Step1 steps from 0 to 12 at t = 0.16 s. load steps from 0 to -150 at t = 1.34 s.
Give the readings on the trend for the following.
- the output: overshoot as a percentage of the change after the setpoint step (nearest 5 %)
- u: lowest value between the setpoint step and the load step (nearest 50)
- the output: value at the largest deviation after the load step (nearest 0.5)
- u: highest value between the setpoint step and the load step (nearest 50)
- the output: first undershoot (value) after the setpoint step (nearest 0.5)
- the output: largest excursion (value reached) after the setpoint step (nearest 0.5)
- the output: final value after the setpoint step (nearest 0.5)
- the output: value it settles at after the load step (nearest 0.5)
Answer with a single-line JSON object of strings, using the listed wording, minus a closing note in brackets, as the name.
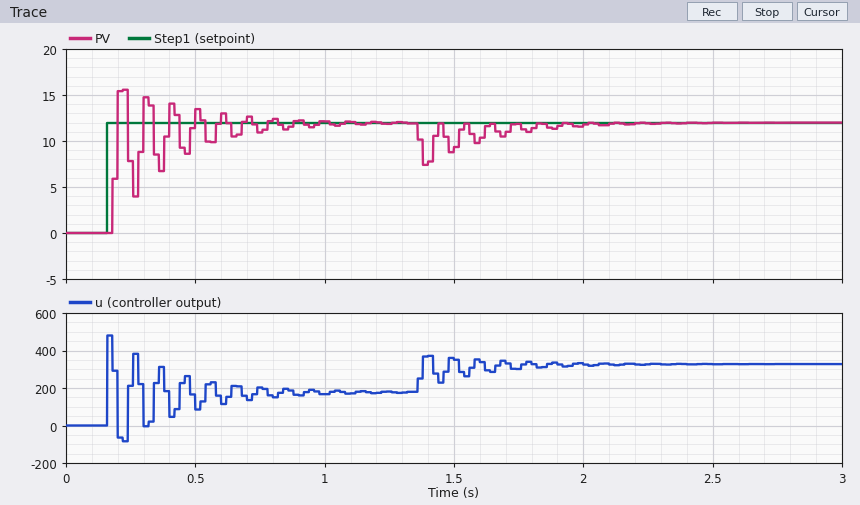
{"the output: overshoot as a percentage of the change after the setpoint step": "30 %", "u: lowest value between the setpoint step and the load step": "-100", "the output: value at the largest deviation after the load step": "7.5", "u: highest value between the setpoint step and the load step": "500", "the output: first undershoot (value) after the setpoint step": "4.0", "the output: largest excursion (value reached) after the setpoint step": "15.5", "the output: final value after the setpoint step": "12.0", "the output: value it settles at after the load step": "12.0"}
